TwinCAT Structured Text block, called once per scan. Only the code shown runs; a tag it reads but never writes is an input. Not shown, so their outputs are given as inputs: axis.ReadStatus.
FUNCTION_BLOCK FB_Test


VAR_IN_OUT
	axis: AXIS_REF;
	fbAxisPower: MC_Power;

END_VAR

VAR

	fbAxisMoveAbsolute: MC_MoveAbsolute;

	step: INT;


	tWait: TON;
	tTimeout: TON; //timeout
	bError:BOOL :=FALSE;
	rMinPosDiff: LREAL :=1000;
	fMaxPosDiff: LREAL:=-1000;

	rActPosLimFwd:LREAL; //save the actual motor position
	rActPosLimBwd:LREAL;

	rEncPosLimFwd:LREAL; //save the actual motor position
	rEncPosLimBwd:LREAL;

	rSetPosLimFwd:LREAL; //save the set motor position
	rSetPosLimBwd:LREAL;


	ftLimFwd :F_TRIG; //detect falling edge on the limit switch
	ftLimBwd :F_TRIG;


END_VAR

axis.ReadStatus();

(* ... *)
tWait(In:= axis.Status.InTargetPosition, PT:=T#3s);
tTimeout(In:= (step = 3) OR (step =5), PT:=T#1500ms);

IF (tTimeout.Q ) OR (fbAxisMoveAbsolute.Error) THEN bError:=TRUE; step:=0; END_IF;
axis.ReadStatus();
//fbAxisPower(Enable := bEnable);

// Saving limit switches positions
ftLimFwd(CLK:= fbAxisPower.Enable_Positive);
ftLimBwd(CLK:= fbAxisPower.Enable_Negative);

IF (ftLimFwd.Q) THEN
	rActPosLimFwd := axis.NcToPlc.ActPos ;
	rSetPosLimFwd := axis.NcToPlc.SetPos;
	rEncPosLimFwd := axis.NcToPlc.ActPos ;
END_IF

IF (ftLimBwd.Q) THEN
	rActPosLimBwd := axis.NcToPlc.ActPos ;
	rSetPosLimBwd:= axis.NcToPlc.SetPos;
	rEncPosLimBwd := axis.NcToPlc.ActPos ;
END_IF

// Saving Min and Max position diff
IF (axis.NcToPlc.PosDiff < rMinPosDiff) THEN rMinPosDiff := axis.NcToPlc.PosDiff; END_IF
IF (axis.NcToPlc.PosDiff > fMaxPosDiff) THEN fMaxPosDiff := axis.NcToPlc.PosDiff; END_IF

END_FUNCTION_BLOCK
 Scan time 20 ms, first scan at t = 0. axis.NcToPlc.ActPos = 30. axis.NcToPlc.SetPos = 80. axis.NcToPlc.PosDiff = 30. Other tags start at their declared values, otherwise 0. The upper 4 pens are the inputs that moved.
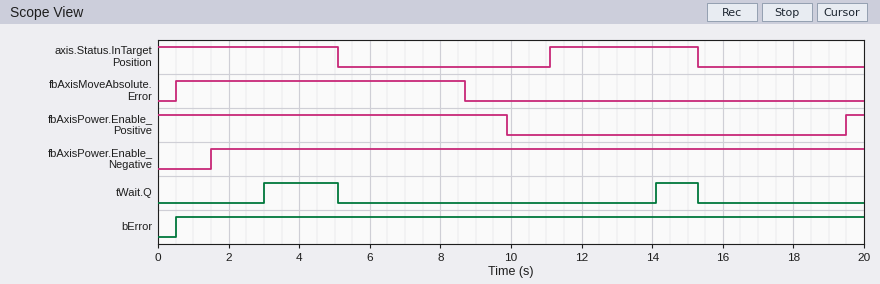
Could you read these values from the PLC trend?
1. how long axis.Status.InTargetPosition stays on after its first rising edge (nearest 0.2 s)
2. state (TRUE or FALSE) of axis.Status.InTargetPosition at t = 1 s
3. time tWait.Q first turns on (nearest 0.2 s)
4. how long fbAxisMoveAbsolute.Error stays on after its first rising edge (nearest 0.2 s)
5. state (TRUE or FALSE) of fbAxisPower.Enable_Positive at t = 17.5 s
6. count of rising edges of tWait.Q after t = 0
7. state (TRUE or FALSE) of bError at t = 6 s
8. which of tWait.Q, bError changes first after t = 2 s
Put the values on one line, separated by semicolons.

4.2 s; TRUE; 3.0 s; 8.2 s; FALSE; 2; TRUE; tWait.Q
